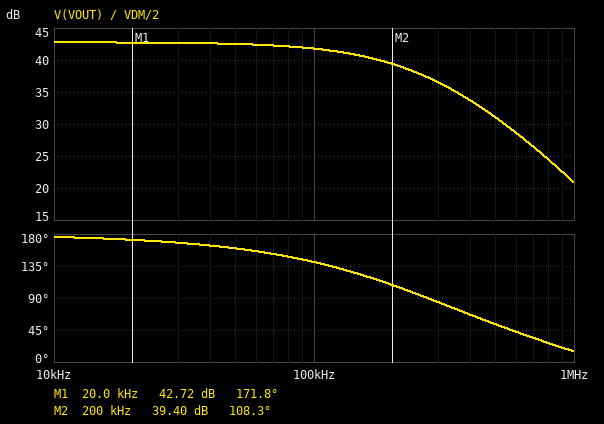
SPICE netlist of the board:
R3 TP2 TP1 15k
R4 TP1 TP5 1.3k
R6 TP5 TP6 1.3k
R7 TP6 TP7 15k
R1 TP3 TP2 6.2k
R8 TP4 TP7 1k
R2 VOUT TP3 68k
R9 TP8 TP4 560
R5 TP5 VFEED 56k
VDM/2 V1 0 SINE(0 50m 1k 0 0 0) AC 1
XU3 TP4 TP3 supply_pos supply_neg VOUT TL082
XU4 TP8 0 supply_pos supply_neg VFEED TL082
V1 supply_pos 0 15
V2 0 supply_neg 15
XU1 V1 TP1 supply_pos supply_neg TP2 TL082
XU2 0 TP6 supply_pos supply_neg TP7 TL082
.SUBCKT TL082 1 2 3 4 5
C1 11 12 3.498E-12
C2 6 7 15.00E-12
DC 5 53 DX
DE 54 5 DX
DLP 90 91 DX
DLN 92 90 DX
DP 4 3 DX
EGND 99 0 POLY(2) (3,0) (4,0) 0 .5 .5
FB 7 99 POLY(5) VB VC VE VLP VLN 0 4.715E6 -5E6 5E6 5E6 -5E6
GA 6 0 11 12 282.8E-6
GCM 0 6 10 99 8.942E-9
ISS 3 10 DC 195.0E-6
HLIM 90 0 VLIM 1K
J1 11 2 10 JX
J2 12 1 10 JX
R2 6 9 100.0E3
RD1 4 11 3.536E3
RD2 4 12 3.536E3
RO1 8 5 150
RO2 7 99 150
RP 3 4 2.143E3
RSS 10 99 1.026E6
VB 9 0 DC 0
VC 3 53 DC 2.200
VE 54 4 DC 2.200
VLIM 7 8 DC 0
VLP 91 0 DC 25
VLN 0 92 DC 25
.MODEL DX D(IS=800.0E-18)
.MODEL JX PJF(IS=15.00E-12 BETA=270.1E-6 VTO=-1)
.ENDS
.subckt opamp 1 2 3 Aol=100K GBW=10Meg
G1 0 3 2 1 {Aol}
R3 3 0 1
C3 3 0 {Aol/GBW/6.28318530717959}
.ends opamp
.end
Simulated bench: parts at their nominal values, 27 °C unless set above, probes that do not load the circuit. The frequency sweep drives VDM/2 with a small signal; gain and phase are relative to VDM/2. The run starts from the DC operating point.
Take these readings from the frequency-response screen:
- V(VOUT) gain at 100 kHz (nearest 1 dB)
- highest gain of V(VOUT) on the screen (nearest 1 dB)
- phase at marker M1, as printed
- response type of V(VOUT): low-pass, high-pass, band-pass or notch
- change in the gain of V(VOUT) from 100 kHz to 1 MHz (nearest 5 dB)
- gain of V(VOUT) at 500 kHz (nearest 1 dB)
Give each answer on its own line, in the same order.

42 dB
43 dB
171.8 deg
low-pass
-20 dB
31 dB
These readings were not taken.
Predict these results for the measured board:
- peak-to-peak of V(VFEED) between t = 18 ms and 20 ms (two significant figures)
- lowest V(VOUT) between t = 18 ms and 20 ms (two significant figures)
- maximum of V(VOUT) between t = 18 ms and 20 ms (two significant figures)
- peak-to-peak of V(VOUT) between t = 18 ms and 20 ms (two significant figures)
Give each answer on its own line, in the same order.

4.3 V
-6.9 V
6.9 V
14 V
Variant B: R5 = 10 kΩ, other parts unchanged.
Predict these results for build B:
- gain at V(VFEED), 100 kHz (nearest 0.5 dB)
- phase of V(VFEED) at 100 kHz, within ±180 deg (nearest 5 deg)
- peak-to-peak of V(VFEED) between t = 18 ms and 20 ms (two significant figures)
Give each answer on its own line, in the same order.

17.0 dB
155 deg
770 mV
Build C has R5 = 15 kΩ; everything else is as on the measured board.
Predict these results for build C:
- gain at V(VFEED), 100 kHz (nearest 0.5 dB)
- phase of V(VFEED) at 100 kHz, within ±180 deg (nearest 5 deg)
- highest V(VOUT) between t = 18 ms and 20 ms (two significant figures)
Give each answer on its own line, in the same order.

20.5 dB
155 deg
6.9 V
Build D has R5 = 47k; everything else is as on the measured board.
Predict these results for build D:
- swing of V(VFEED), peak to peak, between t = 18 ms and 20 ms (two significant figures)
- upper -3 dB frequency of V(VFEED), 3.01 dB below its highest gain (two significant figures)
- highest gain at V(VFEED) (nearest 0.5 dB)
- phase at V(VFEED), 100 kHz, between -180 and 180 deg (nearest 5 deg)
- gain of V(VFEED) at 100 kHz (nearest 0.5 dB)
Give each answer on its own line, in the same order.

3.6 V
250 kHz
31.0 dB
150 deg
30.5 dB
